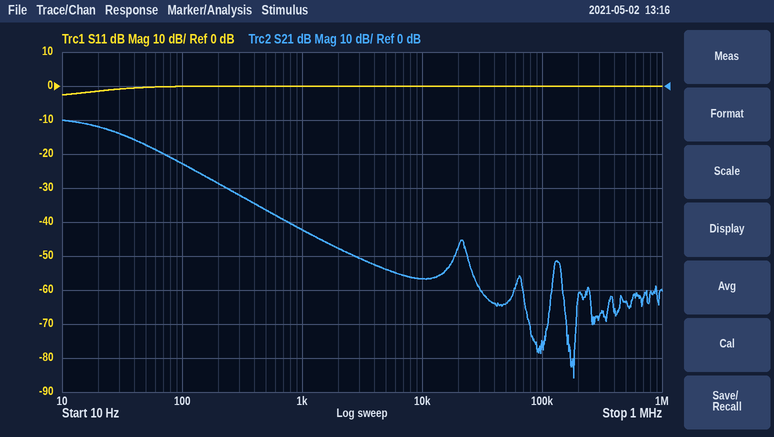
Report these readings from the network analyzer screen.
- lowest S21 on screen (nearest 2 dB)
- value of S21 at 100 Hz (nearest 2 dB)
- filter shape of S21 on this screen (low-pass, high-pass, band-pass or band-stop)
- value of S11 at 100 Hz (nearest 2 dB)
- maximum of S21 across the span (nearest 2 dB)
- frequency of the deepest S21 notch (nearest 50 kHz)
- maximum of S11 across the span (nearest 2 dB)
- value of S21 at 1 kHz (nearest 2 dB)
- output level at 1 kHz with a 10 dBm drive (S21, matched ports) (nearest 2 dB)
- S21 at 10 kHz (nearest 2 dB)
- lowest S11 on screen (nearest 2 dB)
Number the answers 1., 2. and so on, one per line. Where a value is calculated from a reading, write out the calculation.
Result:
1. -86 dB
2. -22 dB
3. low-pass
4. 0 dB
5. -10 dB
6. 200 kHz
7. 0 dB
8. -42 dB
9. 10 dBm + (-42 dB) = -32 dBm
10. -56 dB
11. -2 dB
